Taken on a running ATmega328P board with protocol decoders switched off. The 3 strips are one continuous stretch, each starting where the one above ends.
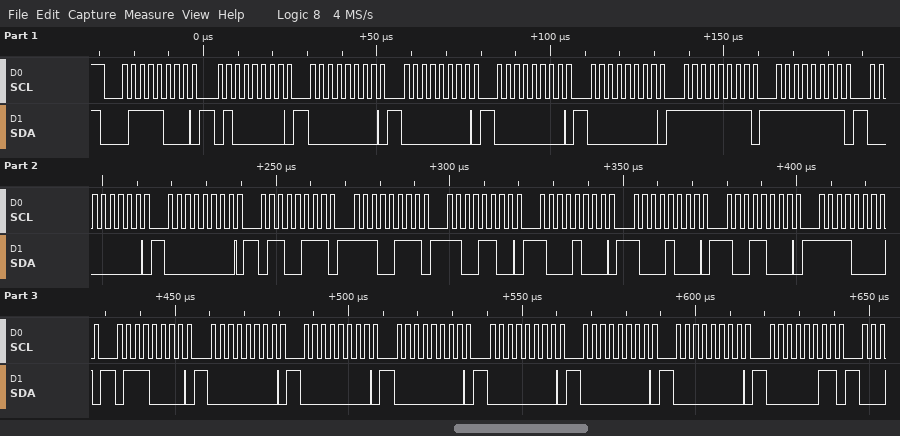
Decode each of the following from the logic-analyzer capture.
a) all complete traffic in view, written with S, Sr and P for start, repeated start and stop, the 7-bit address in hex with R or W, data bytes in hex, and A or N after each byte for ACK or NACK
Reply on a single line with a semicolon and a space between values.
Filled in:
S 3CW A 40 A 00 A 00 A 00 A 00 A FF A FF A 00 A 00 A 67 A E7 A CC A 88 A 88 A 98 A F0 A 70 A 00 A 00 A 00 A 00 A 00 A 00 A 03 A
